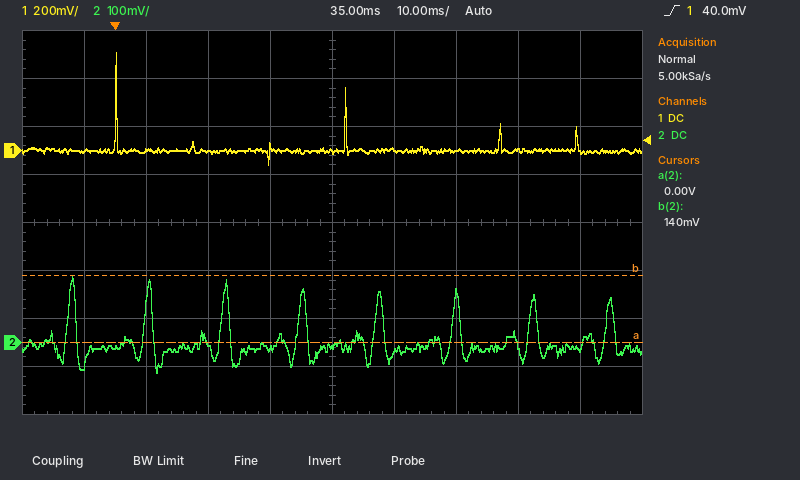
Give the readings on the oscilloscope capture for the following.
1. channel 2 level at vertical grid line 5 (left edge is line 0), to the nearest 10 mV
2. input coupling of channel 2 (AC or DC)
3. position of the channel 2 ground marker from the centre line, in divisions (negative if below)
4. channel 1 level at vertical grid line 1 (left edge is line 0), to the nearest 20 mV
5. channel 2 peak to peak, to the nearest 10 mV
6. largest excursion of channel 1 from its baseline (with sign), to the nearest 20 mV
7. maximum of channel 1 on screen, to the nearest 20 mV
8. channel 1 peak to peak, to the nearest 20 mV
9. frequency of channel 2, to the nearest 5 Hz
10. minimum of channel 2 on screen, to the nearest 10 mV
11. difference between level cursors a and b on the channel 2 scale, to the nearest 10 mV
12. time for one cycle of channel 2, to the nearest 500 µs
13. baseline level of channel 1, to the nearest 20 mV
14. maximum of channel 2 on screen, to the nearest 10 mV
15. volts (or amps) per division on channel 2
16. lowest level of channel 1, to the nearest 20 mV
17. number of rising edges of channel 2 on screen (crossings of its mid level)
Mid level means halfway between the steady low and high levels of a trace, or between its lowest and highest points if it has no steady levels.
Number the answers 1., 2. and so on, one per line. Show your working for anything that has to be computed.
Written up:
1. -10 mV
2. DC
3. -2.5 div
4. 0 mV
5. 140 mV − (-60 mV) = 200 mV
6. 400 mV − (0 mV) = +400 mV
7. 400 mV
8. 400 mV − (-60 mV) = 460 mV
9. 1 / 12.5 ms ≈ 80 Hz
10. -60 mV
11. 140 mV
12. 12.5 ms
13. 0 mV
14. 140 mV
15. 100 mV
16. -60 mV
17. 8
